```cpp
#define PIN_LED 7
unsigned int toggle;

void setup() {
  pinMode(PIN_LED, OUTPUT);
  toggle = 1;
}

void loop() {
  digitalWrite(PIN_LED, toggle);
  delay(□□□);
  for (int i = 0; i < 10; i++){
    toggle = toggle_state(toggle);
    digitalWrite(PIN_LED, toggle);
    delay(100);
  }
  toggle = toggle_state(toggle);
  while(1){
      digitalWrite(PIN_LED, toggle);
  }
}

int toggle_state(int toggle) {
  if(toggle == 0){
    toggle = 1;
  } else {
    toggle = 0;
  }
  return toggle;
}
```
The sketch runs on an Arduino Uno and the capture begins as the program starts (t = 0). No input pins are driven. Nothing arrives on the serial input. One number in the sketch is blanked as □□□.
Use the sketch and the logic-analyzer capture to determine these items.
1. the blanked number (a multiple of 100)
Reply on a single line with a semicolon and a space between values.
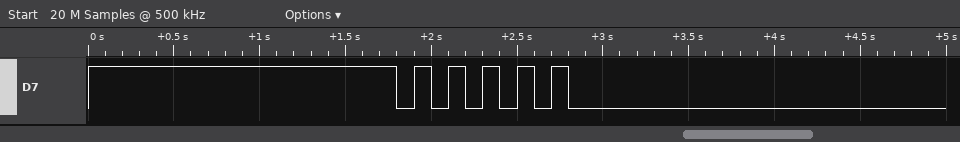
1800
